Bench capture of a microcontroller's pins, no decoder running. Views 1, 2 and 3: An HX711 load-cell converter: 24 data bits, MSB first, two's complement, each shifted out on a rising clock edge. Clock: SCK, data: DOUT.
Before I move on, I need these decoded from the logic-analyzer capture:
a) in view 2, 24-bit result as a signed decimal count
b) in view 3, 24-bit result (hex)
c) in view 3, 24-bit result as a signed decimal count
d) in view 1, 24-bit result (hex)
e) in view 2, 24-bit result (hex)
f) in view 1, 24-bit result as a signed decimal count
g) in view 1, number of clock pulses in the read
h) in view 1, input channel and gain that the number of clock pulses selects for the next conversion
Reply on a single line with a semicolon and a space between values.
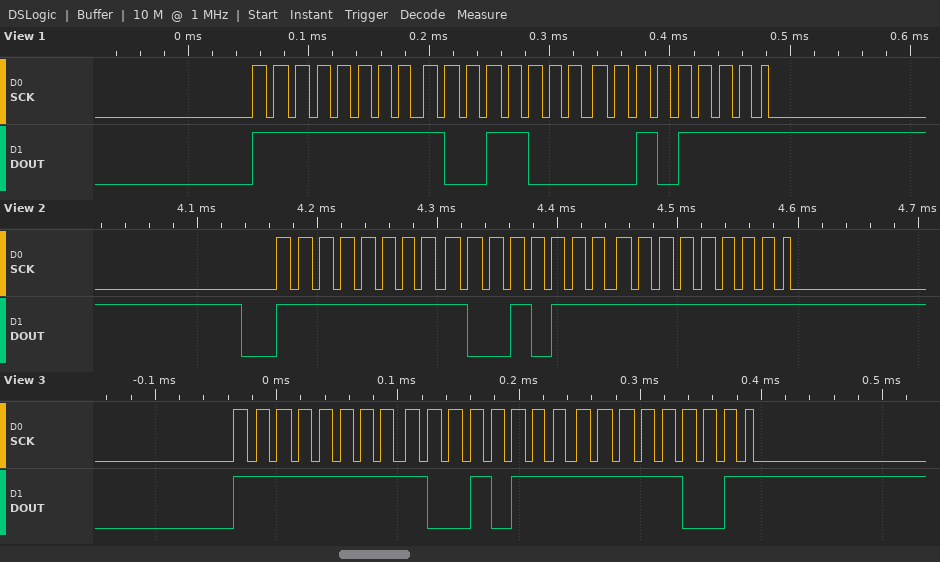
-26625; 0xFF97F9; -26631; 0xFF982F; 0xFF97FF; -26577; 25; channel A, gain 128
